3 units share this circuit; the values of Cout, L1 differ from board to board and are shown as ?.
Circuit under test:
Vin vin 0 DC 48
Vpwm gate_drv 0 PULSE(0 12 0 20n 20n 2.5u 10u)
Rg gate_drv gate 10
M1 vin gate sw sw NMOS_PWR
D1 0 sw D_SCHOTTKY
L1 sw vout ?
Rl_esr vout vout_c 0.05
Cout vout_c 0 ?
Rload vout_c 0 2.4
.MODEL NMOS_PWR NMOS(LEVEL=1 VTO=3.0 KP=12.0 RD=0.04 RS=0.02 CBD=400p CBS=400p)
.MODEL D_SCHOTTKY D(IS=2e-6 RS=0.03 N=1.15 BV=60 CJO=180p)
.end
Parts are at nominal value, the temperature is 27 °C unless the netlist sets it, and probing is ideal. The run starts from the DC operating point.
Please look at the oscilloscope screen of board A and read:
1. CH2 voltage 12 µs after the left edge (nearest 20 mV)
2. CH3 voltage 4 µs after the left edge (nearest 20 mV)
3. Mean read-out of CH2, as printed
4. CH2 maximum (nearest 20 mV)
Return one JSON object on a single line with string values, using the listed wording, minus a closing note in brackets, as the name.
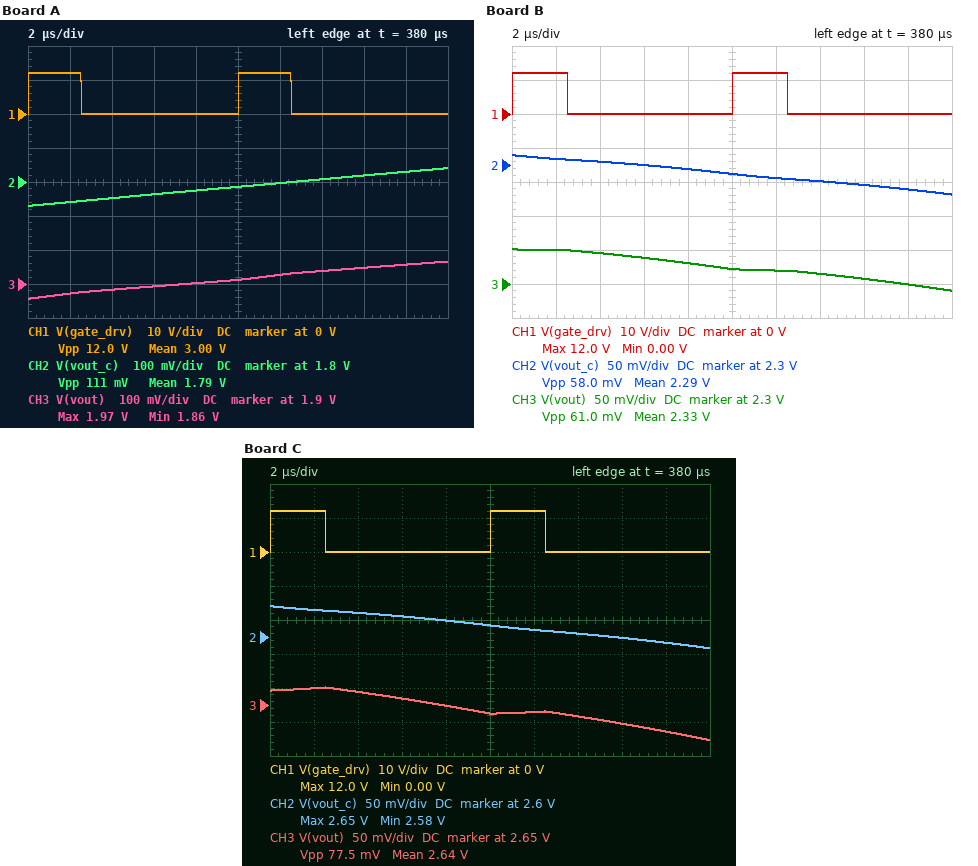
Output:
{"CH2 voltage 12 µs after the left edge": "1.80 V", "CH3 voltage 4 µs after the left edge": "1.88 V", "Mean read-out of CH2, as printed": "1.79 V", "CH2 maximum": "1.84 V"}
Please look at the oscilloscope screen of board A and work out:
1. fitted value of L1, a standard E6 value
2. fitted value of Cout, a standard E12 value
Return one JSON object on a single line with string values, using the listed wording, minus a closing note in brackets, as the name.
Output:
{"fitted value of L1, a standard E6 value": "150 µH", "fitted value of Cout, a standard E12 value": "330 µF"}
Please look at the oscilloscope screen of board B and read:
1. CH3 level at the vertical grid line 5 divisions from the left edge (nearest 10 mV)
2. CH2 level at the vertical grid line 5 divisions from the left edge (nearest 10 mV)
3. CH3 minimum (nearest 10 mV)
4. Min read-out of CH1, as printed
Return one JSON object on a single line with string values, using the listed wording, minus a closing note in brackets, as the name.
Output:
{"CH3 level at the vertical grid line 5 divisions from the left edge": "2.32 V", "CH2 level at the vertical grid line 5 divisions from the left edge": "2.29 V", "CH3 minimum": "2.29 V", "Min read-out of CH1, as printed": "0.00 V"}
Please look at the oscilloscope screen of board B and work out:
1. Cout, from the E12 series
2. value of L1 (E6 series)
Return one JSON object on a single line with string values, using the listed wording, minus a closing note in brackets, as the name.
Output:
{"Cout, from the E12 series": "68 µF", "value of L1": "150 µH"}
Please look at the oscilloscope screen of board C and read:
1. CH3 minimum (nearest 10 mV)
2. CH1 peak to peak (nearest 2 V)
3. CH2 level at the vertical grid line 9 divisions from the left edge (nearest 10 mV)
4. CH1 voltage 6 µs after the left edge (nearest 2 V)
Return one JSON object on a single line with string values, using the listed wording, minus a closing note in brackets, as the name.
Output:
{"CH3 minimum": "2.60 V", "CH1 peak to peak": "12 V", "CH2 level at the vertical grid line 9 divisions from the left edge": "2.59 V", "CH1 voltage 6 µs after the left edge": "0 V"}
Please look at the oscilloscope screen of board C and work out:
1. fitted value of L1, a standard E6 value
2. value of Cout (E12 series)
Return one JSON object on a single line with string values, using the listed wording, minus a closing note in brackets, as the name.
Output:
{"fitted value of L1, a standard E6 value": "68 µH", "value of Cout": "180 µF"}
